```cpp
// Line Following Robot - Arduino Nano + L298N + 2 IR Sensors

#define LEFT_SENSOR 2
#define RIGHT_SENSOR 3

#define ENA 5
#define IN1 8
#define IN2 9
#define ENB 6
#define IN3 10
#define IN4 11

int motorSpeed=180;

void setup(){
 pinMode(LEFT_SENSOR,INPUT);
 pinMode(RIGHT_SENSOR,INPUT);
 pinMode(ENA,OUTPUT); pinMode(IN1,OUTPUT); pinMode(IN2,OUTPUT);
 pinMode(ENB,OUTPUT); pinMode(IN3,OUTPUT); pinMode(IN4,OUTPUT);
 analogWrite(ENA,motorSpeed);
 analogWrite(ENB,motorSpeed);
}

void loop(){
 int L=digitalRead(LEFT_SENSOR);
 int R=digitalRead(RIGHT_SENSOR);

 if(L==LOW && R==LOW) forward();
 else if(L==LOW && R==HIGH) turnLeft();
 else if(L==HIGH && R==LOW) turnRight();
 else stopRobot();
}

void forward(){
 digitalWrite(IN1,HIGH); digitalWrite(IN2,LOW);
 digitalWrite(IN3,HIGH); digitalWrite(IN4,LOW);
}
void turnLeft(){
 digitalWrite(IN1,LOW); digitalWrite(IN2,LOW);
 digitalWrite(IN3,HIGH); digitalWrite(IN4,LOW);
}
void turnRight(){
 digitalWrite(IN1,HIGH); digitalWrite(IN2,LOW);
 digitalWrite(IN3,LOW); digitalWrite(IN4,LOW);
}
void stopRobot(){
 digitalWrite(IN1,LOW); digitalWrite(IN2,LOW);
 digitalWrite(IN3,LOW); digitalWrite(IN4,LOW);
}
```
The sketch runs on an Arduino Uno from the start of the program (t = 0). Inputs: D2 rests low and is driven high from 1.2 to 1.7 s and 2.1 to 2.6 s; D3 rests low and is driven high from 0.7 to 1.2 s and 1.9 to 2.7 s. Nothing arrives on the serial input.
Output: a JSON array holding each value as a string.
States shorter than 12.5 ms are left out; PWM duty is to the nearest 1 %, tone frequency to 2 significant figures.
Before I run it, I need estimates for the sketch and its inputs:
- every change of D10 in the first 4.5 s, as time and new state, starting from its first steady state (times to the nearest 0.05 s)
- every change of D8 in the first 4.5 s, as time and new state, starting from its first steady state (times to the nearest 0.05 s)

["0 s high; 1.2 s low; 1.7 s high; 2.1 s low; 2.6 s high", "0 s high; 0.7 s low; 1.2 s high; 1.9 s low; 2.7 s high"]
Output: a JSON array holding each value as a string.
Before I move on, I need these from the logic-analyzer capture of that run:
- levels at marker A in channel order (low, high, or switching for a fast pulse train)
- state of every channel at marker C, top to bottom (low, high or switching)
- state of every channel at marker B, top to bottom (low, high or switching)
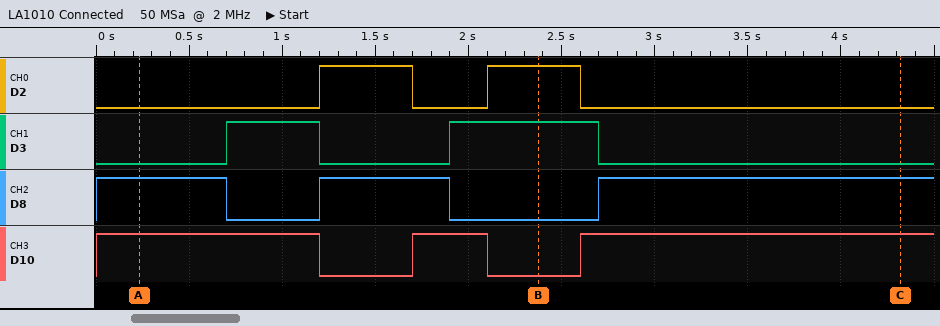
["D2 low, D3 low, D8 high, D10 high", "D2 low, D3 low, D8 high, D10 high", "D2 high, D3 high, D8 low, D10 low"]
